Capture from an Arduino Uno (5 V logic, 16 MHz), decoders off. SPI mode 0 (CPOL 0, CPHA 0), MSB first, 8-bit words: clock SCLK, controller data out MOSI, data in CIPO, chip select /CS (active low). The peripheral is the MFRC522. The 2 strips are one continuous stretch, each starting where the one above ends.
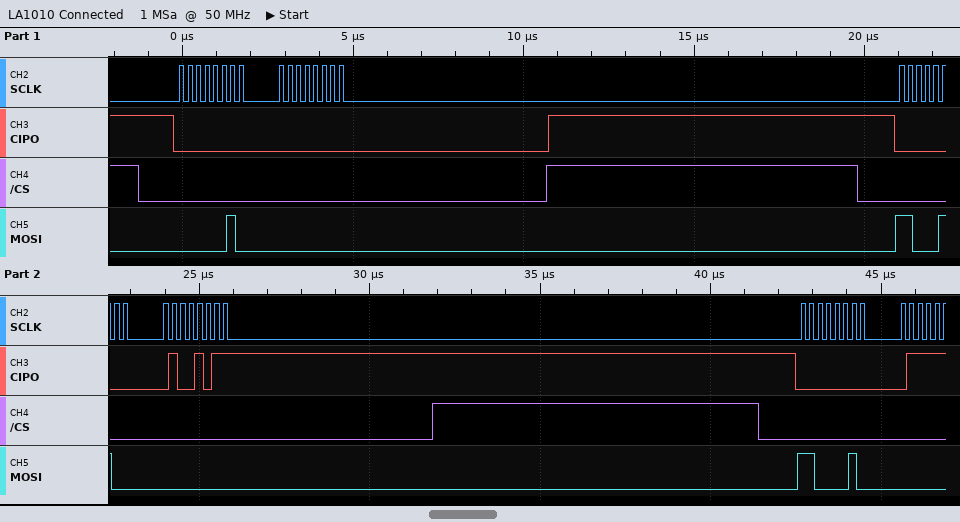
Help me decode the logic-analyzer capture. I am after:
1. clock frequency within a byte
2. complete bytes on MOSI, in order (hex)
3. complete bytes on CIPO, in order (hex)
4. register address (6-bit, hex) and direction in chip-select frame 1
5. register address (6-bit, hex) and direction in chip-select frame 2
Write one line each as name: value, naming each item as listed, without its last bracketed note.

clock frequency within a byte: 4 MHz
complete bytes on MOSI, in order: 02 00 C4 00 C2
complete bytes on CIPO, in order: 00 00 00 4B 00
register address (6-bit, hex) and direction in chip-select frame 1: 0x01 write
register address (6-bit, hex) and direction in chip-select frame 2: 0x22 read
